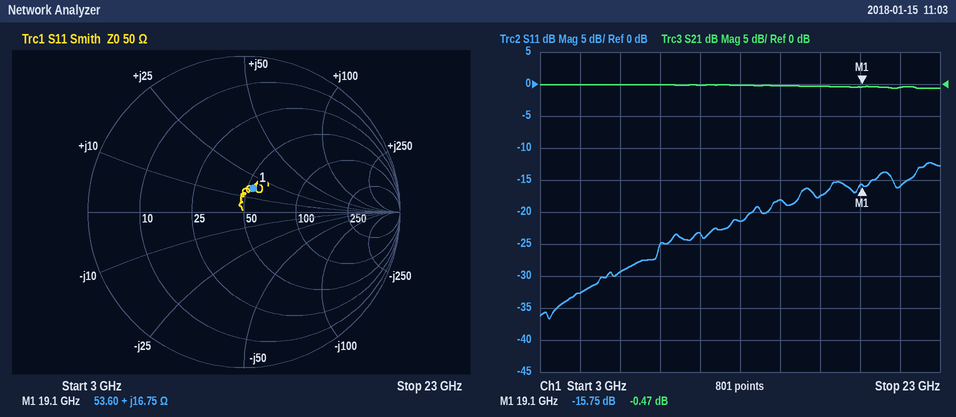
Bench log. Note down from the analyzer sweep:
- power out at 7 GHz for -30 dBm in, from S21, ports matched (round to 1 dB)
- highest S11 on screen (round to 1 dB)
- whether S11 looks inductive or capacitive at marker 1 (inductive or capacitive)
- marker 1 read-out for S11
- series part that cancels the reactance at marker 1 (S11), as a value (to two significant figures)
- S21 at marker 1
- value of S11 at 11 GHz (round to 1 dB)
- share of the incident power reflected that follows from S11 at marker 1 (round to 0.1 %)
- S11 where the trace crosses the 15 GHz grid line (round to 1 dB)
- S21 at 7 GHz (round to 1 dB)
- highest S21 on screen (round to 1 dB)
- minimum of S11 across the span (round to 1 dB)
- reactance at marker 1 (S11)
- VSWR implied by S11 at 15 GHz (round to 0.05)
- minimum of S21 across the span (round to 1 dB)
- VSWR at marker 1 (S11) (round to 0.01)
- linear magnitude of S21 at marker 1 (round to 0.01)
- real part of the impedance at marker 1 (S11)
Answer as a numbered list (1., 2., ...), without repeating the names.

1. -30 dBm
2. -12 dB
3. inductive
4. -15.75 dB
5. 500 fF
6. -0.47 dB
7. -23 dB
8. 2.7 %
9. -18 dB
10. 0 dB
11. 0 dB
12. -37 dB
13. +16.75 Ω
14. 1.30
15. -1 dB
16. 1.39
17. 0.95
18. 53.60 Ω
